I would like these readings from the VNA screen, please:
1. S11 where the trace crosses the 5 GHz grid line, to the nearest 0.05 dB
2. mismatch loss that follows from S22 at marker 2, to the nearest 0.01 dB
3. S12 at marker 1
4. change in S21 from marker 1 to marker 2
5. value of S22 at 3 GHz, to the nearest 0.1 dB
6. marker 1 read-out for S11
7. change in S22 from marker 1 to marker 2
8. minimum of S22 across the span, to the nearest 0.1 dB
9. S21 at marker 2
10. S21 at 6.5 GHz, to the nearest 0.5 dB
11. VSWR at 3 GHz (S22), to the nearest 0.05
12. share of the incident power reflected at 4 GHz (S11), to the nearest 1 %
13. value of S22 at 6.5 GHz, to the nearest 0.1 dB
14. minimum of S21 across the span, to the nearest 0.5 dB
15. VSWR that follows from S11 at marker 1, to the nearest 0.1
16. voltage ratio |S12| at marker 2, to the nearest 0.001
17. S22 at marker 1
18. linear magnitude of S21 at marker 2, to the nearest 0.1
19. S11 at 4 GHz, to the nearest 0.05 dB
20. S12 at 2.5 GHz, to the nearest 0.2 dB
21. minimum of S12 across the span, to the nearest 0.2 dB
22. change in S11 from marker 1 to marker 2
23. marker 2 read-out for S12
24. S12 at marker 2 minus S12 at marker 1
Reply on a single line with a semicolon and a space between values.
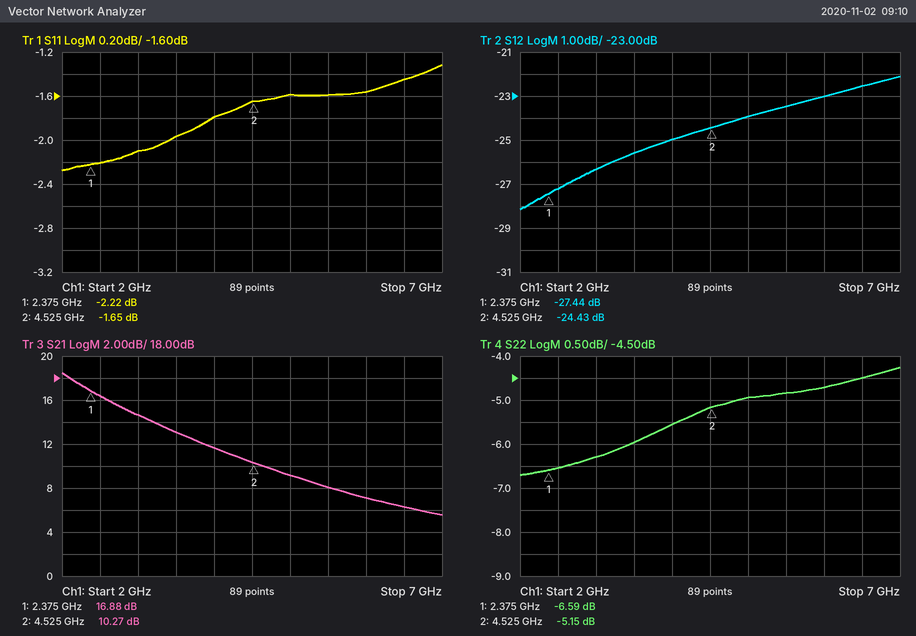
-1.60 dB; 1.58 dB; -27.44 dB; -6.61 dB; -6.3 dB; -2.22 dB; 1.44 dB; -6.7 dB; 10.27 dB; 6.5 dB; 2.90; 66 %; -4.5 dB; 5.5 dB; 7.9; 0.060; -6.59 dB; 3.3; -1.80 dB; -27.2 dB; -28.2 dB; 0.57 dB; -24.43 dB; 3.01 dB
